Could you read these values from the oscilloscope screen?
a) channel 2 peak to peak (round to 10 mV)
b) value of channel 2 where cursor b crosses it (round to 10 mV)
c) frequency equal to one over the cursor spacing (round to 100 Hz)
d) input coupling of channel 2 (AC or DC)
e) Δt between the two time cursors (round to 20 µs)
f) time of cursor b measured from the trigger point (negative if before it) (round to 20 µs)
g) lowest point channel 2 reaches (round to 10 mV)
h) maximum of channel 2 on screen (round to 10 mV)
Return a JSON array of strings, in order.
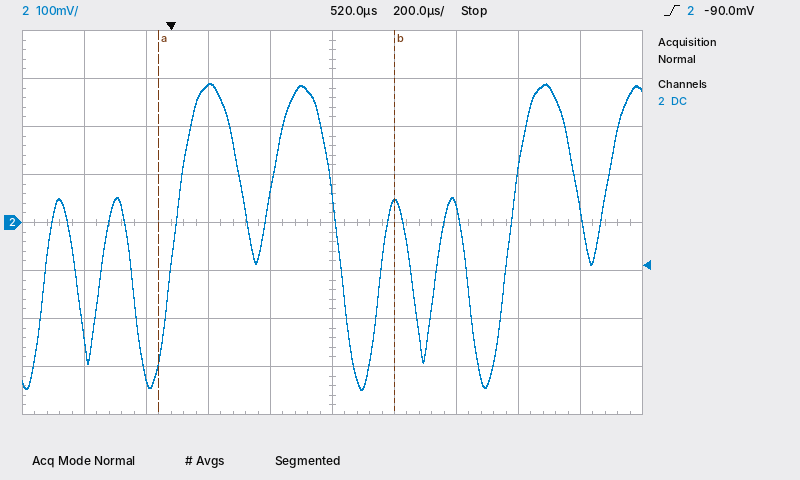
["640 mV", "40 mV", "1.3 kHz", "DC", "760 µs", "+720 µs", "-350 mV", "290 mV"]
